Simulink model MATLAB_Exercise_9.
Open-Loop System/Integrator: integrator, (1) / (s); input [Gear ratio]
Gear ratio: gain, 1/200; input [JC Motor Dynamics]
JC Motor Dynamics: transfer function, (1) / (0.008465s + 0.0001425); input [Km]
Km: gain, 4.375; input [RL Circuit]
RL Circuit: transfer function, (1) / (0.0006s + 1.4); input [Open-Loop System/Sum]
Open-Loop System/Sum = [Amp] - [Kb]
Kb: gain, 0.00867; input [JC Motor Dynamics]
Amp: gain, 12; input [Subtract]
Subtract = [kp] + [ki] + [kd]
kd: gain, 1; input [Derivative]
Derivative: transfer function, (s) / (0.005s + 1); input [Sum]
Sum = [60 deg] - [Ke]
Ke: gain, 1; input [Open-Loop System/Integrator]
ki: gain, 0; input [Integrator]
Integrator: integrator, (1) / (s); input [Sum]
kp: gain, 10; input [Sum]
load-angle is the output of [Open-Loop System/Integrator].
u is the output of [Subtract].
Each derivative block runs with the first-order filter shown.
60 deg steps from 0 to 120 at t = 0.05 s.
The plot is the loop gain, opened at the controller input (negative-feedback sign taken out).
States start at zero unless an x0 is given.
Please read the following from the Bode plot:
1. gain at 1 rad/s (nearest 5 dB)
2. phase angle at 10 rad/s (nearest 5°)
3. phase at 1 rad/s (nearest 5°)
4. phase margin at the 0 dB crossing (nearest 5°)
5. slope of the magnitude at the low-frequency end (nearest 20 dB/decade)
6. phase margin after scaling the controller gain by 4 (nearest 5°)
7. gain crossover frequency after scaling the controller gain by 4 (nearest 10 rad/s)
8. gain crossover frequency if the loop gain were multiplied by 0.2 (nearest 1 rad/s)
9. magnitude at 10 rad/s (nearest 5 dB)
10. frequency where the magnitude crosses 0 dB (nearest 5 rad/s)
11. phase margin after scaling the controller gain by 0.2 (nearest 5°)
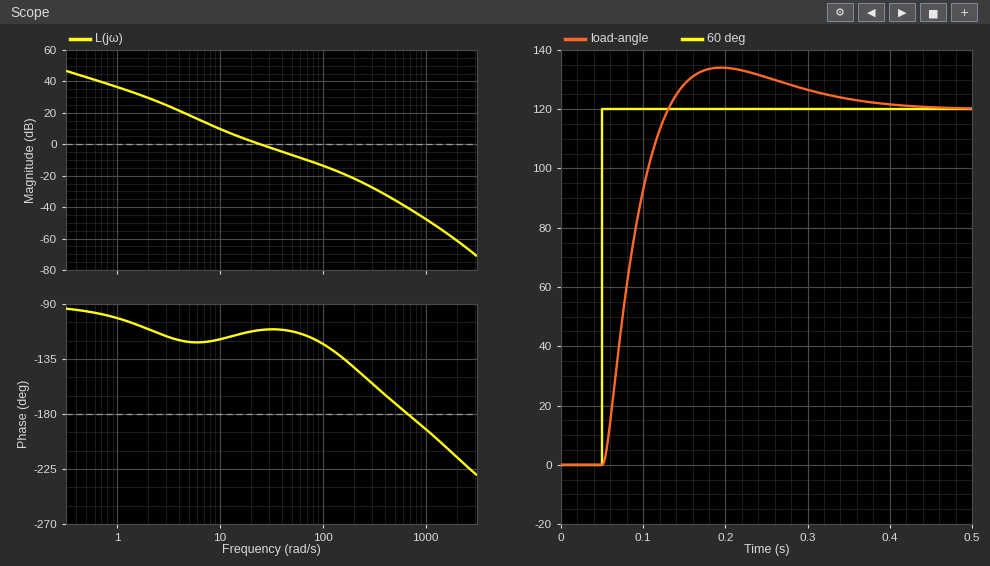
35 dB
-120°
-100°
70°
-20 dB/decade
60°
90 rad/s
7 rad/s
10 dB
25 rad/s
60°
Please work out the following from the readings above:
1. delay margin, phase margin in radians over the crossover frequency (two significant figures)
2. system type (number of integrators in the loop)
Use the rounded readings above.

0.049 s
1
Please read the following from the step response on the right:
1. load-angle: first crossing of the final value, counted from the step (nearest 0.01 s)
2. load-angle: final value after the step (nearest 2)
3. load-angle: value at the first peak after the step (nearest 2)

0.08 s
120
134
